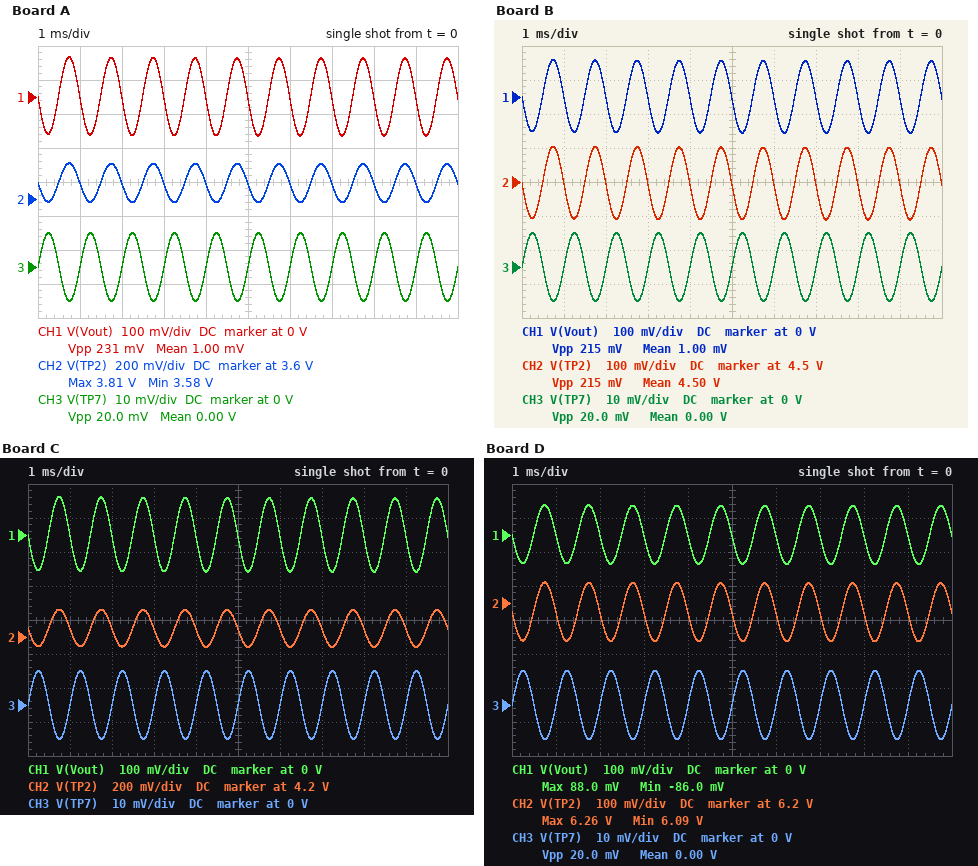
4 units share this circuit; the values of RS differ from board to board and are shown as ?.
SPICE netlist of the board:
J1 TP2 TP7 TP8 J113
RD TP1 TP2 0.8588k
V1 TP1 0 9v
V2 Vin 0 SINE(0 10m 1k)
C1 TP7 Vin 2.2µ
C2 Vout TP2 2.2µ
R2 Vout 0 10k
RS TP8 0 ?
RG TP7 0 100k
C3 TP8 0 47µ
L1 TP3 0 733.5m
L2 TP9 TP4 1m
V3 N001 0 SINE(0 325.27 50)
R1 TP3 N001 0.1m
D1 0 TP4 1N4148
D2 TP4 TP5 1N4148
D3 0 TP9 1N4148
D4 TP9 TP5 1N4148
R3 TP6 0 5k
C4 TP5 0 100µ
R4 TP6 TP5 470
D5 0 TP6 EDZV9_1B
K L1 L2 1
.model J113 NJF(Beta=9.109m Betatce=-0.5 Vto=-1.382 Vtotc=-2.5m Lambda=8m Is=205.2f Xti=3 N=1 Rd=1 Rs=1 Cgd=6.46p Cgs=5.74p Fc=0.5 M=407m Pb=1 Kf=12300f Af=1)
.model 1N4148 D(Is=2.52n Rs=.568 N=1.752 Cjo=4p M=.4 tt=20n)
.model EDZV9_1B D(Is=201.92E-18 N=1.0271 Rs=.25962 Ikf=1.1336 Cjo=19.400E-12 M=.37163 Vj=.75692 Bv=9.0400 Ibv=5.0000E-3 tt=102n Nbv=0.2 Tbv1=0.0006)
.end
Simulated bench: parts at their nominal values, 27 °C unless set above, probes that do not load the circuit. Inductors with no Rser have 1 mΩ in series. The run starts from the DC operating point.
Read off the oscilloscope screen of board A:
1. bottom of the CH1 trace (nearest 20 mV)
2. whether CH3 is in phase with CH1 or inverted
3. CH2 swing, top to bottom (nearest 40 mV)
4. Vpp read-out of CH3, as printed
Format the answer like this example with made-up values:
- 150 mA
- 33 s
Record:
- -120 mV
- inverted
- 240 mV
- 20.0 mV
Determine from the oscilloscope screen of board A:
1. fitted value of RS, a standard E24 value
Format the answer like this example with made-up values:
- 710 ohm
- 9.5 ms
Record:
- 91 Ω
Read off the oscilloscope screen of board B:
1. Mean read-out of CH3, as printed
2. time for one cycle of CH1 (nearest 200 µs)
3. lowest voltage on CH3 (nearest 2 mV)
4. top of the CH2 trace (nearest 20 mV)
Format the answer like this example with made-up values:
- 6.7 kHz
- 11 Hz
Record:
- 0.00 V
- 1.0 ms
- -10 mV
- 4.60 V
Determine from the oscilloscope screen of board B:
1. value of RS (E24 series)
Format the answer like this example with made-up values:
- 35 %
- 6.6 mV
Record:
- 120 Ω
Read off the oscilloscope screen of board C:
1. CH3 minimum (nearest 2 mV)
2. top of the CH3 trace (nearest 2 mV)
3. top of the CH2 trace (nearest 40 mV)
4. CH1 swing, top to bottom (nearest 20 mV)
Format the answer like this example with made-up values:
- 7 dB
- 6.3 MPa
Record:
- -10 mV
- 10 mV
- 4.36 V
- 220 mV
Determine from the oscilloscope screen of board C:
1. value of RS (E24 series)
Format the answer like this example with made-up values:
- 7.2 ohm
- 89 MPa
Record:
- 110 Ω
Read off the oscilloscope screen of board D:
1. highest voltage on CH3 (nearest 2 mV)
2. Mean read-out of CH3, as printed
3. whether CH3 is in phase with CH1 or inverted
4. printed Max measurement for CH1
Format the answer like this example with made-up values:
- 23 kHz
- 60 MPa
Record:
- 10 mV
- 0.00 V
- inverted
- 88.0 mV
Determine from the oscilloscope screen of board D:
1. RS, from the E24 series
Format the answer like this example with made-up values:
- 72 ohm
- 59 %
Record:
- 240 Ω
